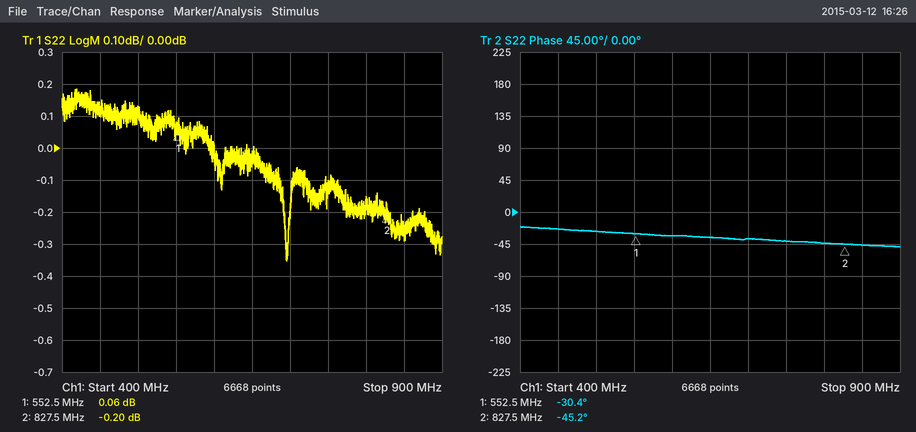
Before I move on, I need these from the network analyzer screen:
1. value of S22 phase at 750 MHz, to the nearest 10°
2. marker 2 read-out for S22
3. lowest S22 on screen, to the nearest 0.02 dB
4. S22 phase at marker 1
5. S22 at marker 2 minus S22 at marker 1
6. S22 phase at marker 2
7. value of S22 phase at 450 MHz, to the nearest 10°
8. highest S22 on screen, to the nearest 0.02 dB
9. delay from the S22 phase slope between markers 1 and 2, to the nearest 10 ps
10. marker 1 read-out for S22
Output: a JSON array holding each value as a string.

["-40°", "-0.20 dB", "-0.36 dB", "-30.4°", "-0.26 dB", "-45.2°", "-20°", "0.18 dB", "150 ps", "0.06 dB"]
